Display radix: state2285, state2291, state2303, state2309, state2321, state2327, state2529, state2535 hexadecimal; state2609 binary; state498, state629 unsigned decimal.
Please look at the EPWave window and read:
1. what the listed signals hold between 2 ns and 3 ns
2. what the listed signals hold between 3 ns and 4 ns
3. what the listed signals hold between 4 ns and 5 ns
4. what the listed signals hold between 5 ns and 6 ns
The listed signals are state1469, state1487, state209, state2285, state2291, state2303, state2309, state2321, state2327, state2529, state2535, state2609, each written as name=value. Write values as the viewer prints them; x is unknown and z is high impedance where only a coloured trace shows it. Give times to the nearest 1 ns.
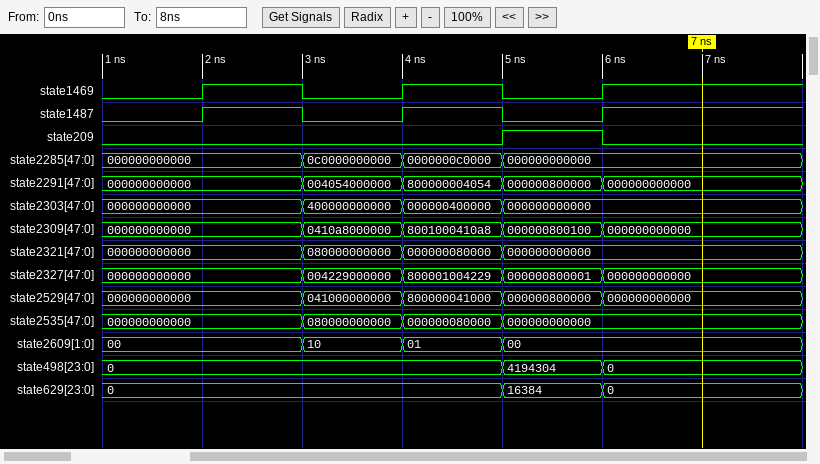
state1469=1, state1487=1, state209=0, state2285=000000000000, state2291=000000000000, state2303=000000000000, state2309=000000000000, state2321=000000000000, state2327=000000000000, state2529=000000000000, state2535=000000000000, state2609=00
state1469=0, state1487=0, state209=0, state2285=0c0000000000, state2291=004054000000, state2303=400000000000, state2309=0410a8000000, state2321=080000000000, state2327=004229000000, state2529=041000000000, state2535=080000000000, state2609=10
state1469=1, state1487=1, state209=0, state2285=0000000c0000, state2291=800000004054, state2303=000000400000, state2309=8001000410a8, state2321=000000080000, state2327=800001004229, state2529=800000041000, state2535=000000080000, state2609=01
state1469=0, state1487=0, state209=1, state2285=000000000000, state2291=000000800000, state2303=000000000000, state2309=000000800100, state2321=000000000000, state2327=000000800001, state2529=000000800000, state2535=000000000000, state2609=00
